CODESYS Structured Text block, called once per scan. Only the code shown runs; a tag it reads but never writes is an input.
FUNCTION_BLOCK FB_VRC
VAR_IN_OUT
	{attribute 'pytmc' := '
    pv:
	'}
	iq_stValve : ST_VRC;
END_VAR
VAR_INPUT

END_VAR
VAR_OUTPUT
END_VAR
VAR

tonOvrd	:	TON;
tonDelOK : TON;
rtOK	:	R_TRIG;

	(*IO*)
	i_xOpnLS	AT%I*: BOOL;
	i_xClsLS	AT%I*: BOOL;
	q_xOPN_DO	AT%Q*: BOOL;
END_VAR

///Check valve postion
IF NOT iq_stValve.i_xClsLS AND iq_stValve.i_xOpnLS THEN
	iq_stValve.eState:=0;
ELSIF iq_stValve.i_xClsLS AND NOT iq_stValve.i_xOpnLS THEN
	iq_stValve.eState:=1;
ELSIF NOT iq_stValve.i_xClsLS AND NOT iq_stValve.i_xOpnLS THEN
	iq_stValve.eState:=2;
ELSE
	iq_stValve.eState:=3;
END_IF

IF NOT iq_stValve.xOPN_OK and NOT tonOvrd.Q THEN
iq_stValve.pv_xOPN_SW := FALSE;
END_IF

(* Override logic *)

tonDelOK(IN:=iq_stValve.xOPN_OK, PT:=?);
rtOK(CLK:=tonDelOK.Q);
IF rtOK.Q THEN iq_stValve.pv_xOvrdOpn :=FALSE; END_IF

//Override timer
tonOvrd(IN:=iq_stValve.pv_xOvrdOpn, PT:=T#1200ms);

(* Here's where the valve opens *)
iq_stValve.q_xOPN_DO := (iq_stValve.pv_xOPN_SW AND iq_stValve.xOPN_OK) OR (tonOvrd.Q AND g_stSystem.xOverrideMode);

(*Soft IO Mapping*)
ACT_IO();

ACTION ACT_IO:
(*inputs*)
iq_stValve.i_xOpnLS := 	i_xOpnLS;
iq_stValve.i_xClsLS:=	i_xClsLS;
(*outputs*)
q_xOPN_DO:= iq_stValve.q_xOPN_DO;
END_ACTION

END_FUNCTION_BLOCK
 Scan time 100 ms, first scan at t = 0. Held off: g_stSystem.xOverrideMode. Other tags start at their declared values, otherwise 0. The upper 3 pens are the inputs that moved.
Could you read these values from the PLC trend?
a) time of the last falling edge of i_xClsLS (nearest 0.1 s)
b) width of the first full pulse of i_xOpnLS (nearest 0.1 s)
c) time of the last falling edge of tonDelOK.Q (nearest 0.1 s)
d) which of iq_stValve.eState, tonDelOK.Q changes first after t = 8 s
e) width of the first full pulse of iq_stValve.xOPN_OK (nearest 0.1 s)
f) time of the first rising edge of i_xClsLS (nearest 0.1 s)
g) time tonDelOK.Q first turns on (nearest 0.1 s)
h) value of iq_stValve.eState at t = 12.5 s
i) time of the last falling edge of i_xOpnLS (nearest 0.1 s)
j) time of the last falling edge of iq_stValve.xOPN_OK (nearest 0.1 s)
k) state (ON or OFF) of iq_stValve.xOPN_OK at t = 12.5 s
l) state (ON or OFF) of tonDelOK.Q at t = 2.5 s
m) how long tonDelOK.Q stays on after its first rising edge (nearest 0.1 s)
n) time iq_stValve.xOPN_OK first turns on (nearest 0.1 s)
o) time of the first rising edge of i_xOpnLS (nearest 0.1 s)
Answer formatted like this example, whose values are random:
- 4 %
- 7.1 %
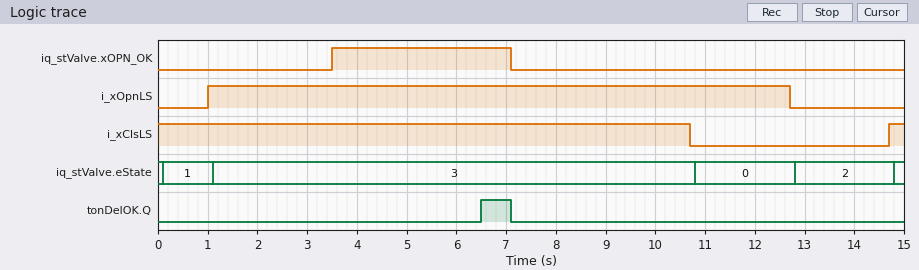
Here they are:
- 10.7 s
- 11.7 s
- 7.1 s
- iq_stValve.eState
- 3.6 s
- 14.7 s
- 6.5 s
- 0
- 12.7 s
- 7.1 s
- OFF
- OFF
- 0.6 s
- 3.5 s
- 1.0 s
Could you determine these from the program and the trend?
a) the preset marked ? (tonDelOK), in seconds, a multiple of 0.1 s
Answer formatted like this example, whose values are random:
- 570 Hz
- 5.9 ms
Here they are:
- 3.0 s
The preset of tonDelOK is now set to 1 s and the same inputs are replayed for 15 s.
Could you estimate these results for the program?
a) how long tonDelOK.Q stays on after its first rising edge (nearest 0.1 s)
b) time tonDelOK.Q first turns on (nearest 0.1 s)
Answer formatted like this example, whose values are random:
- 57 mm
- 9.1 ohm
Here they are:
- 2.6 s
- 4.5 s
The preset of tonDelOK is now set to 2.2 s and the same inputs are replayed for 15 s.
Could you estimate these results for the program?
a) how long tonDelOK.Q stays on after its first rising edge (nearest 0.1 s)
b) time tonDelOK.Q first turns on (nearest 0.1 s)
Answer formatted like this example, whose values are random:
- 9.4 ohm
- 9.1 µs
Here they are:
- 1.4 s
- 5.7 s
